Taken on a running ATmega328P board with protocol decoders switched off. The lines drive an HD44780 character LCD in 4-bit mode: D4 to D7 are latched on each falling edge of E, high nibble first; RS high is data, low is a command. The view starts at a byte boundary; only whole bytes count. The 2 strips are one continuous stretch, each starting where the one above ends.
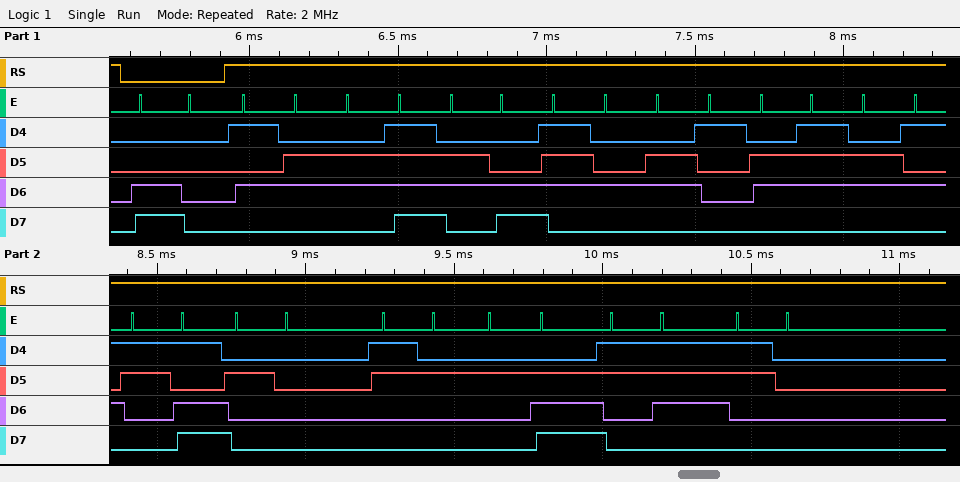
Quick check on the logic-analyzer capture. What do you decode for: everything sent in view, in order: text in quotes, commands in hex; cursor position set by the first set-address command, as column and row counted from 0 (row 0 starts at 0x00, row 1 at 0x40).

0xC0 "Voltage= 2.70"
column 0, row 1
